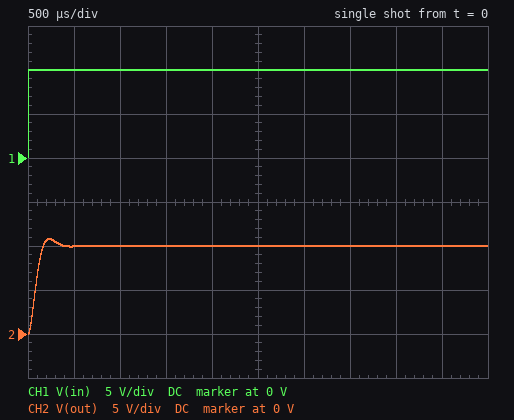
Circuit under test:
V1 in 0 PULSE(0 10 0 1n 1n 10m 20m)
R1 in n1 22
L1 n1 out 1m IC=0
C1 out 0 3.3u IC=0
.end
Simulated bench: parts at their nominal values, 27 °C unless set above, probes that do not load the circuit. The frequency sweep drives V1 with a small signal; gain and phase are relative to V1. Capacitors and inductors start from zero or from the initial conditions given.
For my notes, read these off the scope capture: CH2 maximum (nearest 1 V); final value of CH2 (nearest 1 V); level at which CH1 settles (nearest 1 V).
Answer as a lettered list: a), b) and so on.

a) 11 V
b) 10 V
c) 10 V
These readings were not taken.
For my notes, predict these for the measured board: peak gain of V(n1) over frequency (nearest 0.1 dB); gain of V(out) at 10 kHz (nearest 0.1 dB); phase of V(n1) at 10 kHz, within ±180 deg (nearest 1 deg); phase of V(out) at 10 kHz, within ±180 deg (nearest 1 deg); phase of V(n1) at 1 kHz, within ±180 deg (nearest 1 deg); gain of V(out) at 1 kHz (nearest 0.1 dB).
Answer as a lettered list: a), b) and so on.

a) 0 dB
b) -22.2 dB
c) 21 deg
d) -159 deg
e) -28 deg
f) 0.2 dB
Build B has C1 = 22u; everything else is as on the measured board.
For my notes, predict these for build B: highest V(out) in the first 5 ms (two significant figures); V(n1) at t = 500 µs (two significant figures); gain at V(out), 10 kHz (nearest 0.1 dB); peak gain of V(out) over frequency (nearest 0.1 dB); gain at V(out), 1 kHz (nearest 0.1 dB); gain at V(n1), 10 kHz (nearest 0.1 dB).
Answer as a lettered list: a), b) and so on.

a) 10 V
b) 6.0 V
c) -39.2 dB
d) 0 dB
e) -9.7 dB
f) -0.5 dB
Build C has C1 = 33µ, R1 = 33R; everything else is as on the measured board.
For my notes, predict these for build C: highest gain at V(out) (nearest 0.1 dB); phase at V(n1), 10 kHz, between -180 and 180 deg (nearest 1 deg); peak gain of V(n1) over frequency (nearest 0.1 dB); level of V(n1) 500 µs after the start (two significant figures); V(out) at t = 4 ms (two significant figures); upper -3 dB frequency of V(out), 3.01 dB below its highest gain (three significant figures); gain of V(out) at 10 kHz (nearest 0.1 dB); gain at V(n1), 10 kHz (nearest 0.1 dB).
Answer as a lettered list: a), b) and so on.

a) 0 dB
b) 28 deg
c) 0 dB
d) 3.4 V
e) 9.8 V
f) 150 Hz
g) -43.3 dB
h) -1.1 dB
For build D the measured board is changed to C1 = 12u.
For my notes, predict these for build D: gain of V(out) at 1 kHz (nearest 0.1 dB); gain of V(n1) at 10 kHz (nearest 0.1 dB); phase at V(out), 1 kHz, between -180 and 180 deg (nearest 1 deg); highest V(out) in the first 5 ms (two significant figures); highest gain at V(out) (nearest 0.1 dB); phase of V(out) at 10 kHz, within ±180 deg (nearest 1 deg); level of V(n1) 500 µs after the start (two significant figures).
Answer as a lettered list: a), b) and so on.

a) -4.8 dB
b) -0.5 dB
c) -72 deg
d) 10 V
e) 0 dB
f) -160 deg
g) 8.4 V
